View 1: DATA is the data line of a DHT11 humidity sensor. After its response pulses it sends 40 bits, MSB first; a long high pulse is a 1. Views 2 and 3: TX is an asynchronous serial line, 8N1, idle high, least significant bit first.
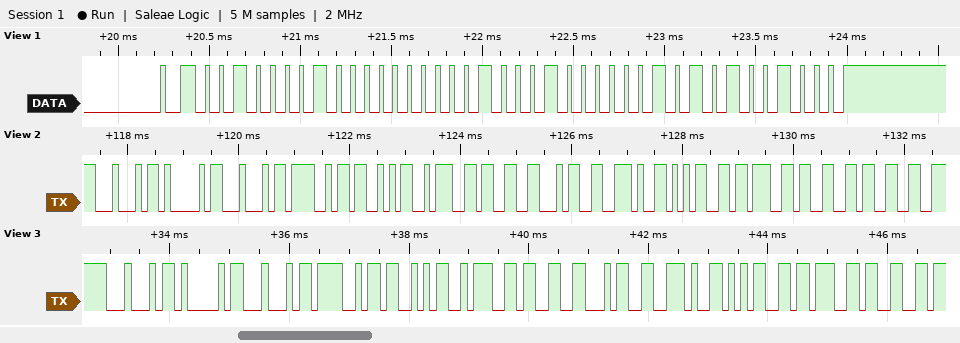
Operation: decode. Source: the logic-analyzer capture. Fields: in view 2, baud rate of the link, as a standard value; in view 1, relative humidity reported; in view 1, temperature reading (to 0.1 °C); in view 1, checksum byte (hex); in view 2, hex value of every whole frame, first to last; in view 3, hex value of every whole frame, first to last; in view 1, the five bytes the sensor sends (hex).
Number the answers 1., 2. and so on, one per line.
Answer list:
1. 9600 baud
2. 33 %
3. 34.5 °C
4. 0x48
5. 44 41 44 4F 53 3A 33 34 2E 35 3B 33 33
6. 44 41 44 4F 53 3A 33 34 2E 35 3B 33
7. 21 00 22 05 48
